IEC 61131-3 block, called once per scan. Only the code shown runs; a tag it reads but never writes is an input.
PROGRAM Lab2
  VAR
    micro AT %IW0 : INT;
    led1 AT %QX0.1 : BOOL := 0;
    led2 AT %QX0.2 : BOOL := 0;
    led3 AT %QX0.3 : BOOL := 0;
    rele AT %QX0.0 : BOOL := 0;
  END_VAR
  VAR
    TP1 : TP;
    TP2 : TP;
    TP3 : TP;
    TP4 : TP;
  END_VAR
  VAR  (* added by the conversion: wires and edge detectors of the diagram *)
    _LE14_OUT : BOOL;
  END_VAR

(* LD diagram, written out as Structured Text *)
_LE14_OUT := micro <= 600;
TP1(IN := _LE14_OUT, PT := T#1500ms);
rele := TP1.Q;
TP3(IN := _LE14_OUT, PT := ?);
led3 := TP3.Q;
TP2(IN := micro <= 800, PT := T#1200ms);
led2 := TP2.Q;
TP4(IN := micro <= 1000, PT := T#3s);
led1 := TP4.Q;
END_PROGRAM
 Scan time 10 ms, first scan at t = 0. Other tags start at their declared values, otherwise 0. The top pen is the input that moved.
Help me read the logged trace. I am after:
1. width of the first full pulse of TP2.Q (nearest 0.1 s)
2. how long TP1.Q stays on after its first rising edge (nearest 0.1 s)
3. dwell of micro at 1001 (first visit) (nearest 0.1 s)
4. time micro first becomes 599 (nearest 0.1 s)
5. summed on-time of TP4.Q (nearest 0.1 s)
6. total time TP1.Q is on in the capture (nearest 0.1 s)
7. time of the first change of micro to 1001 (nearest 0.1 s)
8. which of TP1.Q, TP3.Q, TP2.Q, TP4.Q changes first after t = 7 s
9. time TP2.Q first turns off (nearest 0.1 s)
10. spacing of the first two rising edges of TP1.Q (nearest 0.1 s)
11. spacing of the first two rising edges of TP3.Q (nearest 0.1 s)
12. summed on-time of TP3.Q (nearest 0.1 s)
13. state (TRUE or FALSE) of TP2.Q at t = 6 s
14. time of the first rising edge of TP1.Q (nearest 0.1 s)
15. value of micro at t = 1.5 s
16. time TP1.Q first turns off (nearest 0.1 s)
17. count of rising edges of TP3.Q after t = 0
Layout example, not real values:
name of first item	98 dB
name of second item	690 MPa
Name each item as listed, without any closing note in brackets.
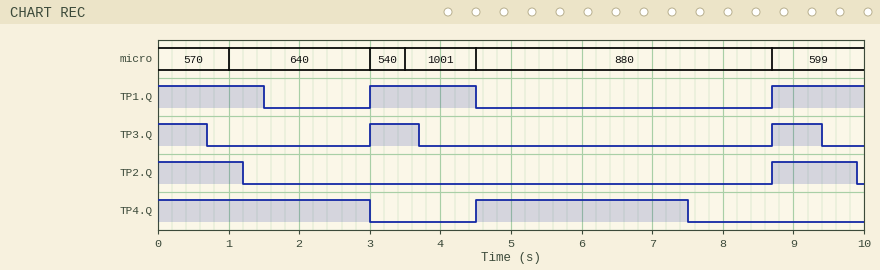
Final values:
width of the first full pulse of TP2.Q	1.2 s
how long TP1.Q stays on after its first rising edge	1.5 s
dwell of micro at 1001 (first visit)	1.0 s
time micro first becomes 599	8.7 s
summed on-time of TP4.Q	6.0 s
total time TP1.Q is on in the capture	4.3 s
time of the first change of micro to 1001	3.5 s
which of TP1.Q, TP3.Q, TP2.Q, TP4.Q changes first after t = 7 s	TP4.Q
time TP2.Q first turns off	1.2 s
spacing of the first two rising edges of TP1.Q	5.7 s
spacing of the first two rising edges of TP3.Q	5.7 s
summed on-time of TP3.Q	2.1 s
state (TRUE or FALSE) of TP2.Q at t = 6 s	FALSE
time of the first rising edge of TP1.Q	3.0 s
value of micro at t = 1.5 s	640
time TP1.Q first turns off	1.5 s
count of rising edges of TP3.Q after t = 0	2
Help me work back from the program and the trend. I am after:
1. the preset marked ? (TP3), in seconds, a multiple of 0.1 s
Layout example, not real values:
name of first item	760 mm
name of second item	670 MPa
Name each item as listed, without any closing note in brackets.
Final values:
the preset marked ? (TP3), in seconds, a multiple of 0.1 s	0.7 s
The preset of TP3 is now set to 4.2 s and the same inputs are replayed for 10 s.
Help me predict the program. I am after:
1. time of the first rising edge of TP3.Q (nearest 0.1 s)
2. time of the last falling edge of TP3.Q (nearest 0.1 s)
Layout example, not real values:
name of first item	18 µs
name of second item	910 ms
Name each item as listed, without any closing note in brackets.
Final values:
time of the first rising edge of TP3.Q	8.7 s
time of the last falling edge of TP3.Q	4.2 s
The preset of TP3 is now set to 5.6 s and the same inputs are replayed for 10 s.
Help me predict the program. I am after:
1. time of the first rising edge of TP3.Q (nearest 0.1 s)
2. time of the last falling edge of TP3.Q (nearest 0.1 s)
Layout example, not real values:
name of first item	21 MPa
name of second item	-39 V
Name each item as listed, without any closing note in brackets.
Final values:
time of the first rising edge of TP3.Q	8.7 s
time of the last falling edge of TP3.Q	5.6 s
